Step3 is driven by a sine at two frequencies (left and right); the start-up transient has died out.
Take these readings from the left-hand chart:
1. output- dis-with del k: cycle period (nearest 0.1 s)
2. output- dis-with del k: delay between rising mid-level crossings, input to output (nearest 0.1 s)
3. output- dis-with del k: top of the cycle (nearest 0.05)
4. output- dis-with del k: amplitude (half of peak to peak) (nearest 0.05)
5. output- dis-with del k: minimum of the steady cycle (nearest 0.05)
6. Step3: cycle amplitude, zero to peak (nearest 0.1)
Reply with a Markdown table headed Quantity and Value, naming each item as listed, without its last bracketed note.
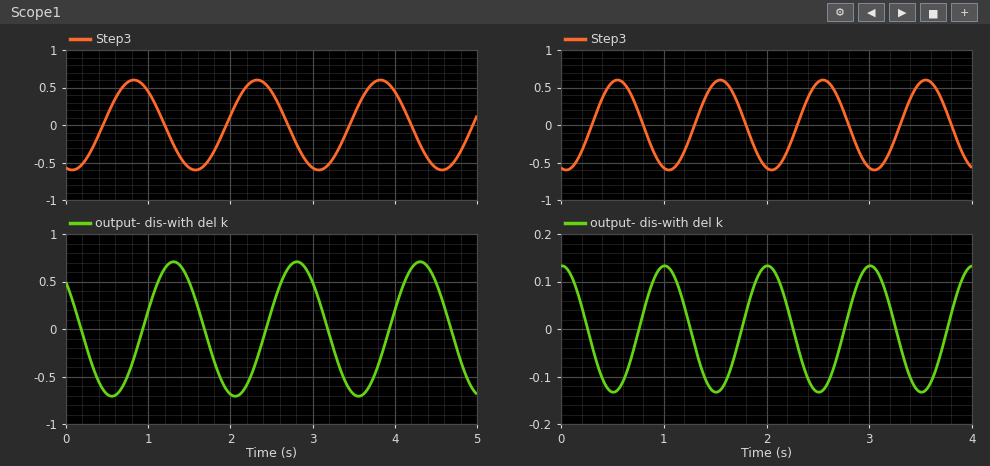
| Quantity | Value |
|---|---|
| output- dis-with del k: cycle period | 1.5 s |
| output- dis-with del k: delay between rising mid-level crossings, input to output | 0.5 s |
| output- dis-with del k: top of the cycle | 0.70 |
| output- dis-with del k: amplitude (half of peak to peak) | 0.70 |
| output- dis-with del k: minimum of the steady cycle | -0.70 |
| Step3: cycle amplitude, zero to peak | 0.6 |
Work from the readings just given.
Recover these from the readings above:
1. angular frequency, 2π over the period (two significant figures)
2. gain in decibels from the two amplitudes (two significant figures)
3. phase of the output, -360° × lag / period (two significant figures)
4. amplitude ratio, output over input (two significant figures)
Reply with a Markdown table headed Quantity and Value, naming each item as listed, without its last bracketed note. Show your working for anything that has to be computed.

| Quantity | Value |
|---|---|
| angular frequency, 2π over the period | 2π / 1.5 = 4.2 rad/s |
| gain in decibels from the two amplitudes | 20 log10(0.7 / 0.6) = 1.3 dB |
| phase of the output, -360° × lag / period | -360 × 0.5 / 1.5 = -120° |
| amplitude ratio, output over input | 0.7 / 0.6 = 1.2 |
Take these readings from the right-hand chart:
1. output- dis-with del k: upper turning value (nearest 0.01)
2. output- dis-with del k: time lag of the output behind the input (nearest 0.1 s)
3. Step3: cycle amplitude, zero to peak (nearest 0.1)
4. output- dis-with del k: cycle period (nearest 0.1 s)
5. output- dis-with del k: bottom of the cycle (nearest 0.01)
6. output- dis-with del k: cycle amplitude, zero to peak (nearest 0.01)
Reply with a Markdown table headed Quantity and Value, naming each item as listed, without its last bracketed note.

| Quantity | Value |
|---|---|
| output- dis-with del k: upper turning value | 0.13 |
| output- dis-with del k: time lag of the output behind the input | 0.5 s |
| Step3: cycle amplitude, zero to peak | 0.6 |
| output- dis-with del k: cycle period | 1.0 s |
| output- dis-with del k: bottom of the cycle | -0.13 |
| output- dis-with del k: cycle amplitude, zero to peak | 0.13 |
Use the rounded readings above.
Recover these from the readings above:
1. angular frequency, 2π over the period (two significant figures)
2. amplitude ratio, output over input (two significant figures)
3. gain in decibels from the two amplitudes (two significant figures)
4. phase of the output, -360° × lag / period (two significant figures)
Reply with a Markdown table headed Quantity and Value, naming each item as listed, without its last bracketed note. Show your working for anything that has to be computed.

| Quantity | Value |
|---|---|
| angular frequency, 2π over the period | 2π / 1 = 6.3 rad/s |
| amplitude ratio, output over input | 0.13 / 0.6 = 0.22 |
| gain in decibels from the two amplitudes | 20 log10(0.13 / 0.6) = -13 dB |
| phase of the output, -360° × lag / period | -360 × 0.5 / 1 = -180° |
